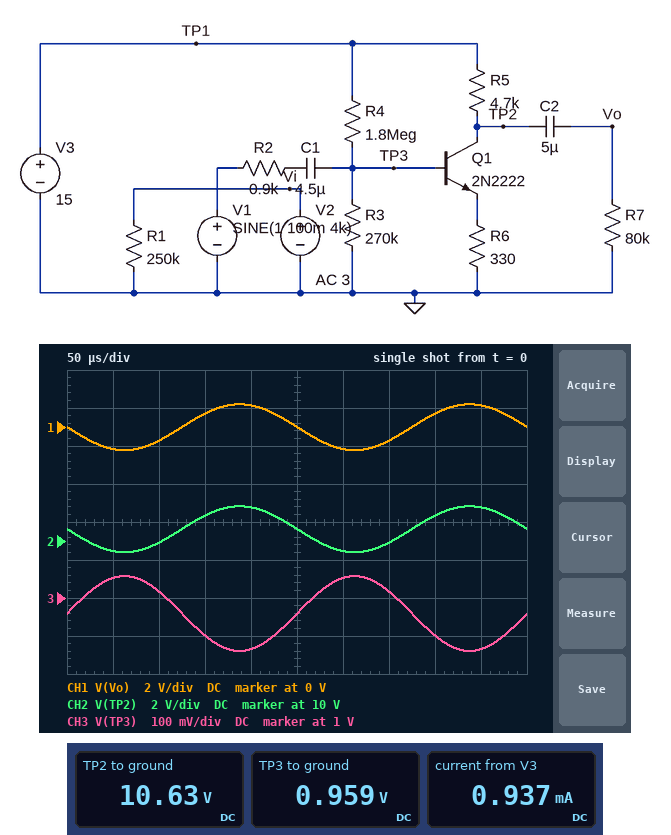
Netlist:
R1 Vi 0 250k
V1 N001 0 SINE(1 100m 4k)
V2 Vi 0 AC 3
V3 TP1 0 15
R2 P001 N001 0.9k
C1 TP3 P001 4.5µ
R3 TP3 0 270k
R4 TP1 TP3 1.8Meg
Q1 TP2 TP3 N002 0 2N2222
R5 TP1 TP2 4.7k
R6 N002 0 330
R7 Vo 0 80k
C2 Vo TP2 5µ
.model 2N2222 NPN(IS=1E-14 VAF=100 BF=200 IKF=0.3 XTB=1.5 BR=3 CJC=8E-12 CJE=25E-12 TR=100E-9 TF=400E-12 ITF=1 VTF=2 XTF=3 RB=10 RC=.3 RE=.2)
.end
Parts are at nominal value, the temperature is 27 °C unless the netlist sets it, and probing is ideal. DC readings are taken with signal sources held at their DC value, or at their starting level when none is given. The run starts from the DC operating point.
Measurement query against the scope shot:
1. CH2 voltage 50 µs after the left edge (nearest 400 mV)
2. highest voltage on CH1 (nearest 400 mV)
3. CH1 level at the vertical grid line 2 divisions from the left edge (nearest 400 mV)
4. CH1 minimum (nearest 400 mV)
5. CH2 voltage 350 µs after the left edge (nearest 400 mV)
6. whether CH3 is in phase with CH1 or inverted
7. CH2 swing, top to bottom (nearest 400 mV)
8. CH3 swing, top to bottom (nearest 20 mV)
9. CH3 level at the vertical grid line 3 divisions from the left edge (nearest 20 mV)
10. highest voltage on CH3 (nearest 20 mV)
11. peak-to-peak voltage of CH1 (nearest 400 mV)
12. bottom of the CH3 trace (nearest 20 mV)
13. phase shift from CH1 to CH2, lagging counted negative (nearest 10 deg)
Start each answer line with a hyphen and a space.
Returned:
- 9.6 V
- 1.2 V
- -800 mV
- -1.2 V
- 10.0 V
- inverted
- 2.4 V
- 200 mV
- 900 mV
- 1.06 V
- 2.4 V
- 860 mV
- 0 deg
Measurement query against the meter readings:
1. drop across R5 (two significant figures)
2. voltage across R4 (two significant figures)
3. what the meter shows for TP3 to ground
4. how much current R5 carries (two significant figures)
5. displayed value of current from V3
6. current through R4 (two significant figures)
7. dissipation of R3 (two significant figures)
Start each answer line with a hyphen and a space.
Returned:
- 4.4 V
- 14 V
- 0.959 V
- 930 µA
- 0.937 mA
- 7.8 µA
- 3.4 µW
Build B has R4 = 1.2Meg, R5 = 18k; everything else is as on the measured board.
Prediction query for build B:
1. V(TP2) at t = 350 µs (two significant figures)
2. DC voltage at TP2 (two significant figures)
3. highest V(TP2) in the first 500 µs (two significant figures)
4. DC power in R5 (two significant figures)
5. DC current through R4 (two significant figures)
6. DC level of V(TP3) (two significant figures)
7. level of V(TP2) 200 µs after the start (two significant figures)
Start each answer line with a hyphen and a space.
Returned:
- 340 mV
- 380 mV
- 4.1 V
- 12 mW
- 12 µA
- 920 mV
- 3.9 V
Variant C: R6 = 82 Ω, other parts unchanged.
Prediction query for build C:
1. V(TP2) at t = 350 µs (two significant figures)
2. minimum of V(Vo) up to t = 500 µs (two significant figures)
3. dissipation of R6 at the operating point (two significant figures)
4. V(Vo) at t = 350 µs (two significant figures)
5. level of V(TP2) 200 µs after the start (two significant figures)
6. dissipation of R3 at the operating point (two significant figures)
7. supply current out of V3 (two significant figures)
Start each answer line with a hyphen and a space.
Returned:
- 7.3 V
- -4.2 V
- 100 µW
- -2.4 V
- 13 V
- 2.1 µW
- 1.1 mA
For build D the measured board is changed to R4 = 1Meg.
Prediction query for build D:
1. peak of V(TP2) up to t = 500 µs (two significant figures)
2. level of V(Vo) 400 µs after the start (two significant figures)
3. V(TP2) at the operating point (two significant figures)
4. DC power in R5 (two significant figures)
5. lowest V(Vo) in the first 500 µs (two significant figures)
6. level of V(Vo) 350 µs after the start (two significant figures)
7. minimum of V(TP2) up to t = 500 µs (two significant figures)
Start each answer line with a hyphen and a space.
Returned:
- 7.5 V
- 740 mV
- 6.2 V
- 16 mW
- -1.3 V
- -740 mV
- 5.0 V
